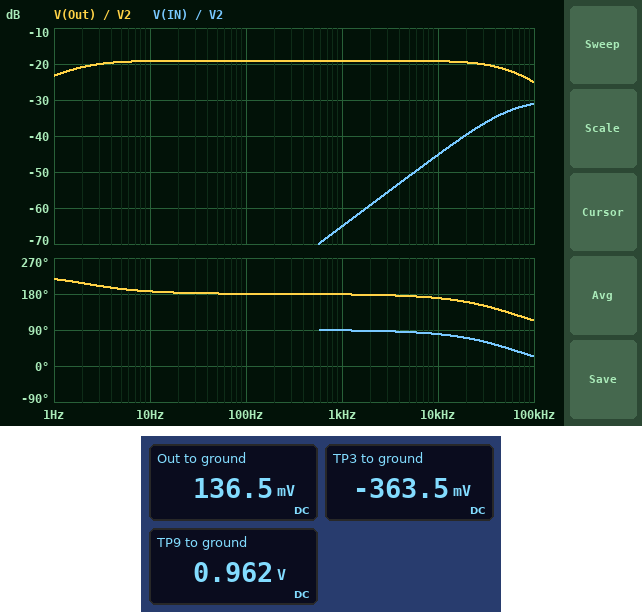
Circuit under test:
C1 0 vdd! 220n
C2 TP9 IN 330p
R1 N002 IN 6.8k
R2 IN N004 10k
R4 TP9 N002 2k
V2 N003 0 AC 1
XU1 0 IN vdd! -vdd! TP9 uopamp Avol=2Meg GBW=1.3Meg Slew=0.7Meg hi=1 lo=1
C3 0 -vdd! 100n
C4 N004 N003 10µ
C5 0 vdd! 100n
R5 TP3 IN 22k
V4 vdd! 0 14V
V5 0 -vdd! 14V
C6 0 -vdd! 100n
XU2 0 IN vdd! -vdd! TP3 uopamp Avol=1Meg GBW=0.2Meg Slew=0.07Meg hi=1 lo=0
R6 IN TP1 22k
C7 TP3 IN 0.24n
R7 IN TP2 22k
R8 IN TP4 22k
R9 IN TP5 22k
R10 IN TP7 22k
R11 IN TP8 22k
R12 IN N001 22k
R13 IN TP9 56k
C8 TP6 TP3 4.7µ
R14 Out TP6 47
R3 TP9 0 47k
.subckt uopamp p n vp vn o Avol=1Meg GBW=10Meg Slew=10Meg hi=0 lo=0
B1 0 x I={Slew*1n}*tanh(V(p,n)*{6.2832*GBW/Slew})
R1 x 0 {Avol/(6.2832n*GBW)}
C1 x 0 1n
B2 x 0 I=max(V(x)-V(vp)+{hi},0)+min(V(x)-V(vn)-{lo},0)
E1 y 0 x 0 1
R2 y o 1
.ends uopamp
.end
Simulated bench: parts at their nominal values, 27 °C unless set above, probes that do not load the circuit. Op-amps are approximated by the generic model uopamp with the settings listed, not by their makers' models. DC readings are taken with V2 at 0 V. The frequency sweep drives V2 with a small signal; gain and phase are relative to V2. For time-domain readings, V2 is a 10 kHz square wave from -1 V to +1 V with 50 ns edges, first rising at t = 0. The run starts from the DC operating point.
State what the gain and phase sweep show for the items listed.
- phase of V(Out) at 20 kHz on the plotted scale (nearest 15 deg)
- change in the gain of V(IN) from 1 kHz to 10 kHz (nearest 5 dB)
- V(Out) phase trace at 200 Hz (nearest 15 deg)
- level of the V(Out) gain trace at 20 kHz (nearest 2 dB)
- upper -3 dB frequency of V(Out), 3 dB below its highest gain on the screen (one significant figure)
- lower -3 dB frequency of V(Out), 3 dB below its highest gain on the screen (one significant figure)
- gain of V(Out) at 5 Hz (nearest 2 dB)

165 deg
20 dB
180 deg
-20 dB
60 kHz
1 Hz
-20 dB
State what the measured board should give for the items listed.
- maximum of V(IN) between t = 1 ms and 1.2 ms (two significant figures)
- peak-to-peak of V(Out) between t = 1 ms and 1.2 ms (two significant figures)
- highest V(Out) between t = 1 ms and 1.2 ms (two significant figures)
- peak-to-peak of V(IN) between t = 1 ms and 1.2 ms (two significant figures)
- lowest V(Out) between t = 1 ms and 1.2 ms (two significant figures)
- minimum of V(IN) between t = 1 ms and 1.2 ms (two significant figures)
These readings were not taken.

61 mV
210 mV
110 mV
120 mV
-99 mV
-61 mV
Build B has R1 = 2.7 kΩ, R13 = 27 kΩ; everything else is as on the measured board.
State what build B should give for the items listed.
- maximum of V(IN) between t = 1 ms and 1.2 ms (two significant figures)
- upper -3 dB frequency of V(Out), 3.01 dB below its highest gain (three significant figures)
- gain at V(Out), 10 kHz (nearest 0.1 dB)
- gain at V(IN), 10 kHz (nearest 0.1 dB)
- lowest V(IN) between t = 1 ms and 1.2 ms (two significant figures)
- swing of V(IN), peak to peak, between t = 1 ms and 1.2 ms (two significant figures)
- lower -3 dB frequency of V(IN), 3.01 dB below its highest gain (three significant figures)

54 mV
110 kHz
-24.5 dB
-50.5 dB
-54 mV
110 mV
89.9 kHz
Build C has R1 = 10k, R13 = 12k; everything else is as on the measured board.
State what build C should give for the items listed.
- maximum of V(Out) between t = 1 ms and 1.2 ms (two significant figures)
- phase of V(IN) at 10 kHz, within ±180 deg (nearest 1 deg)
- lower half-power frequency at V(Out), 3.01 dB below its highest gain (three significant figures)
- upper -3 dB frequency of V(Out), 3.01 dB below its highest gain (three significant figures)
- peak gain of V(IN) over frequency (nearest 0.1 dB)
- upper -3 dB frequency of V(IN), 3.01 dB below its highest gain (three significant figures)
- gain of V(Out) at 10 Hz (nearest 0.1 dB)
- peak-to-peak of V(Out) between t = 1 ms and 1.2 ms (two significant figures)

87 mV
82 deg
1.34 Hz
73.6 kHz
-30.4 dB
988 kHz
-21.1 dB
170 mV
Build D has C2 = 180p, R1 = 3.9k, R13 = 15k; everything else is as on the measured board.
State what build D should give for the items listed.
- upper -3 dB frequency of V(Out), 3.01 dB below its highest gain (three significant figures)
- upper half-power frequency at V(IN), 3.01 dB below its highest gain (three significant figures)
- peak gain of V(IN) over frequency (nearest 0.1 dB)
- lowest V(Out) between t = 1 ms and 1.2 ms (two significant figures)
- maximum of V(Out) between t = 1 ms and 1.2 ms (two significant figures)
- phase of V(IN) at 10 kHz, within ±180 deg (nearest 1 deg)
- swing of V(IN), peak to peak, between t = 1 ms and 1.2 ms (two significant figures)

177 kHz
943 kHz
-26.7 dB
-49 mV
61 mV
86 deg
170 mV
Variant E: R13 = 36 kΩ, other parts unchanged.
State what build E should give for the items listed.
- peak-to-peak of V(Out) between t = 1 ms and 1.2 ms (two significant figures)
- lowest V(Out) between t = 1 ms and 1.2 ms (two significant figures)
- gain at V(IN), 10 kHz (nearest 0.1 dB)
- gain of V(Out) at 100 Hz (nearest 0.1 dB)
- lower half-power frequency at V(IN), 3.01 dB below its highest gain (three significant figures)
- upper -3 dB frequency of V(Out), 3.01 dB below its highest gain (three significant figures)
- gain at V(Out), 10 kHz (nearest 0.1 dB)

190 mV
-92 mV
-45.8 dB
-19.7 dB
55.4 kHz
62.8 kHz
-19.8 dB
